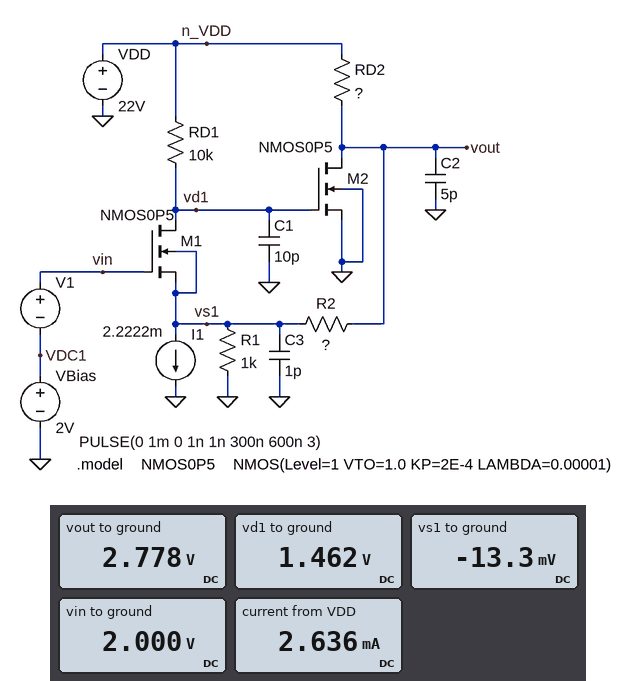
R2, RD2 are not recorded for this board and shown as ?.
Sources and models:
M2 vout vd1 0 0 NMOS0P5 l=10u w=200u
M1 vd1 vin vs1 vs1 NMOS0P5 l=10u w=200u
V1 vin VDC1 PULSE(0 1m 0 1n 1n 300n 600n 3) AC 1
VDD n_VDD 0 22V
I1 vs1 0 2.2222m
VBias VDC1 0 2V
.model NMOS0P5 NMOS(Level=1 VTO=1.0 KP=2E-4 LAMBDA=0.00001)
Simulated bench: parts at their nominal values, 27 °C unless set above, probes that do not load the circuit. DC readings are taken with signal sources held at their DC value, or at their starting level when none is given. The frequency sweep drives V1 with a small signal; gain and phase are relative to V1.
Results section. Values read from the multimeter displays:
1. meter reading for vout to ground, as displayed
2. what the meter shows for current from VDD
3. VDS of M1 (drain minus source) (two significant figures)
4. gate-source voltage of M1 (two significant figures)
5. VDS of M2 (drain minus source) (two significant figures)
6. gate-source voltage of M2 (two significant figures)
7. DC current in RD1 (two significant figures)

2.778 V
2.636 mA
1.5 V
2.0 V
2.8 V
1.5 V
2.1 mA
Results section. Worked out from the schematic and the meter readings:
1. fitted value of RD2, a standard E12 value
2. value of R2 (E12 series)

33 kΩ
18 kΩ
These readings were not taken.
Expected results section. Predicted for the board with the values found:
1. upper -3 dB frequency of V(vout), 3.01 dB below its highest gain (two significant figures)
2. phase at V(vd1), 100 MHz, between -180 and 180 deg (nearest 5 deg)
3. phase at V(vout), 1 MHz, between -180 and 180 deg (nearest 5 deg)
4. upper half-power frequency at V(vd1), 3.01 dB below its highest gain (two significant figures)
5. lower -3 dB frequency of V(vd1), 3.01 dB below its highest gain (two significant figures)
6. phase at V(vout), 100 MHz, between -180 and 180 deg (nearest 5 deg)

8.0 MHz
115 deg
-5 deg
9.0 MHz
4.8 MHz
-145 deg
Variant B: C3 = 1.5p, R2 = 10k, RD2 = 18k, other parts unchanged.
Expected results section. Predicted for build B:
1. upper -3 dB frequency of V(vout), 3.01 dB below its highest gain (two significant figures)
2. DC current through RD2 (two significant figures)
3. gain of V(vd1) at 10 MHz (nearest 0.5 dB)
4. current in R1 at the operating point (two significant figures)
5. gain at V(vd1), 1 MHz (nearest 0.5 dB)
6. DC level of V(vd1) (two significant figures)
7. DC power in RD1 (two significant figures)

13 MHz
1.1 mA
7.5 dB
7.8 µA
-5.0 dB
1.7 V
41 mW
